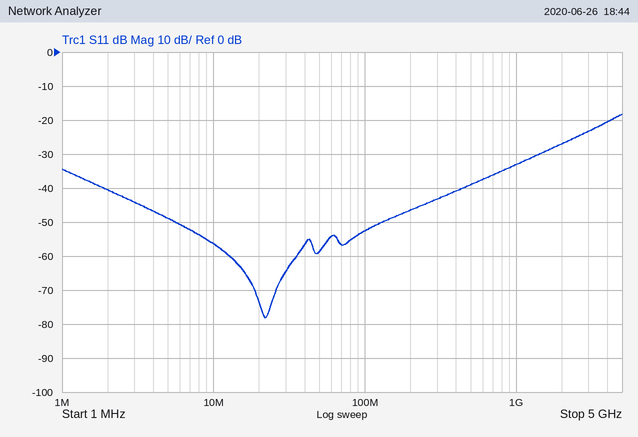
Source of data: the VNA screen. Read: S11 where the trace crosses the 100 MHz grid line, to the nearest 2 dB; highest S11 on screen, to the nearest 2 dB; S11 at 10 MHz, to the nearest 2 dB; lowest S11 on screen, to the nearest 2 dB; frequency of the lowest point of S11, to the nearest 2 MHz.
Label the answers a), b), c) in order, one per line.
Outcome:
a) -52 dB
b) -18 dB
c) -56 dB
d) -78 dB
e) 22 MHz
